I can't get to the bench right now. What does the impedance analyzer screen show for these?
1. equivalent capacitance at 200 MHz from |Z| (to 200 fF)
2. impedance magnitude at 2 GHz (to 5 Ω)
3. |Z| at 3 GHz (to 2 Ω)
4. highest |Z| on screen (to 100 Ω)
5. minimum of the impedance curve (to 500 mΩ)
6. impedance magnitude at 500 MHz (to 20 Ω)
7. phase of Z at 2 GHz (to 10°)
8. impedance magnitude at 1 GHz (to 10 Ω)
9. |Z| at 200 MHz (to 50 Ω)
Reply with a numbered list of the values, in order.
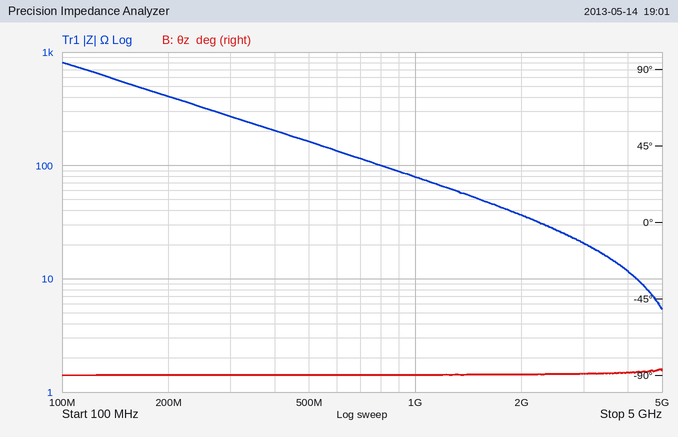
1. 2.0 pF
2. 35 Ω
3. 20 Ω
4. 800 Ω
5. 5.5 Ω
6. 160 Ω
7. -90°
8. 80 Ω
9. 400 Ω
